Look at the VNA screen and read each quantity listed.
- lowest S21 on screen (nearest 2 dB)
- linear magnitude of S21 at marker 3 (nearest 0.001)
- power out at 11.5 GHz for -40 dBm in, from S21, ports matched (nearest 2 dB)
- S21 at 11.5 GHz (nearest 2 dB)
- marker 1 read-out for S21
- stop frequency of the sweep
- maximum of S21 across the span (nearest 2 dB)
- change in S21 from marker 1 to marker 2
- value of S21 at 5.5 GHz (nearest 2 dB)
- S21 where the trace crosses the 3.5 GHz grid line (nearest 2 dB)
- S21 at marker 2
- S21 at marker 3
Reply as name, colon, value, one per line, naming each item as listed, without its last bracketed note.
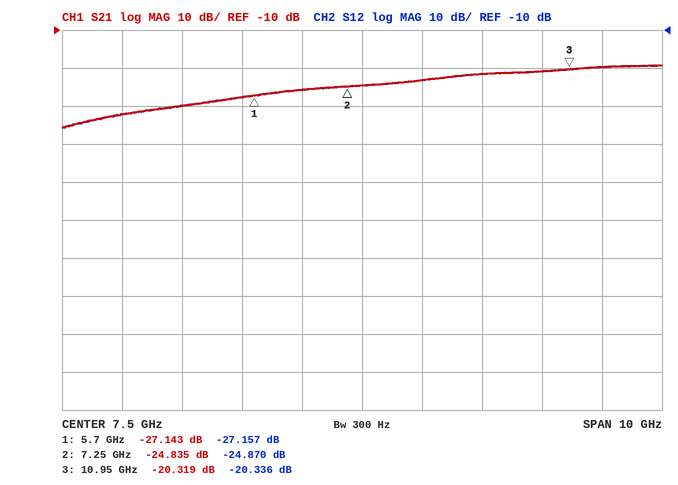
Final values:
lowest S21 on screen: -36 dB
linear magnitude of S21 at marker 3: 0.096
power out at 11.5 GHz for -40 dBm in, from S21, ports matched: -60 dBm
S21 at 11.5 GHz: -20 dB
marker 1 read-out for S21: -27.143 dB
stop frequency of the sweep: 12.5 GHz
maximum of S21 across the span: -20 dB
change in S21 from marker 1 to marker 2: 2.308 dB
value of S21 at 5.5 GHz: -28 dB
S21 where the trace crosses the 3.5 GHz grid line: -32 dB
S21 at marker 2: -24.835 dB
S21 at marker 3: -20.319 dB
